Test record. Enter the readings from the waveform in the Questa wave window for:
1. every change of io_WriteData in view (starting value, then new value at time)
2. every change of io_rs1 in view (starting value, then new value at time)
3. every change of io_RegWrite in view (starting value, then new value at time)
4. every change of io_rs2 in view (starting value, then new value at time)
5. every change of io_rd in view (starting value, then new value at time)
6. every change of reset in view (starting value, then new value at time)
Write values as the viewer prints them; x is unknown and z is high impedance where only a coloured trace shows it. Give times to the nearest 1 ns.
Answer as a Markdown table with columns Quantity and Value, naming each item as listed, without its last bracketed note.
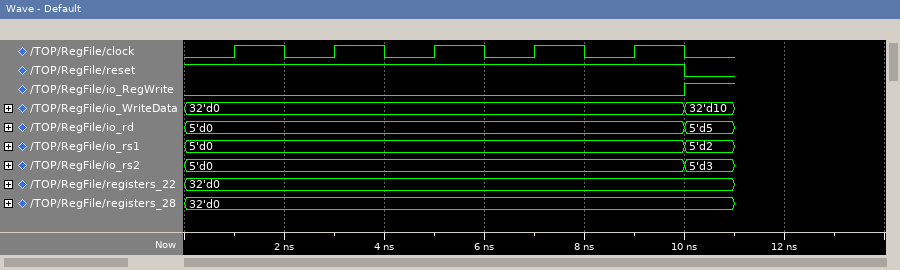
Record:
| Quantity | Value |
|---|---|
| every change of io_WriteData in view | 32'd0, 32'd10 at 10 ns |
| every change of io_rs1 in view | 5'd0, 5'd2 at 10 ns |
| every change of io_RegWrite in view | 0, 1 at 10 ns |
| every change of io_rs2 in view | 5'd0, 5'd3 at 10 ns |
| every change of io_rd in view | 5'd0, 5'd5 at 10 ns |
| every change of reset in view | 1, 0 at 10 ns |
